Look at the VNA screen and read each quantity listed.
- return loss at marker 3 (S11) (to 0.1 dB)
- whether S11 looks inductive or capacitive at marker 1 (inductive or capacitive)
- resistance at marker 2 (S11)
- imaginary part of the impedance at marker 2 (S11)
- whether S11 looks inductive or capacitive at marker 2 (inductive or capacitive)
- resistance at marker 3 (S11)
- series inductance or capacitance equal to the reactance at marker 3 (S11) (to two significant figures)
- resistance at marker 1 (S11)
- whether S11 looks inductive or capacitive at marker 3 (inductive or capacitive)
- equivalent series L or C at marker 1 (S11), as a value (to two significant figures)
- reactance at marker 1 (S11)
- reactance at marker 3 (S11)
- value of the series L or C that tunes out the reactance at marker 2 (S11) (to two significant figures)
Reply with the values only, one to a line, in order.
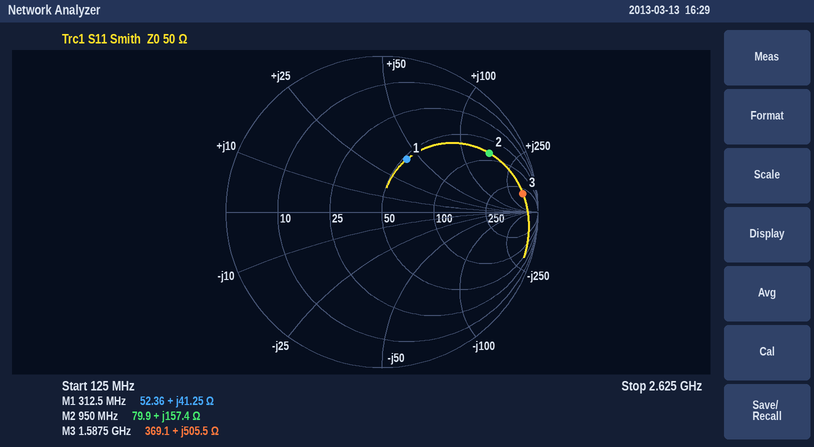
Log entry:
0.8 dB
inductive
79.9 Ω
+157.4 Ω
inductive
369.1 Ω
51 nH
52.36 Ω
inductive
21 nH
+41.25 Ω
+505.5 Ω
1.1 pF
